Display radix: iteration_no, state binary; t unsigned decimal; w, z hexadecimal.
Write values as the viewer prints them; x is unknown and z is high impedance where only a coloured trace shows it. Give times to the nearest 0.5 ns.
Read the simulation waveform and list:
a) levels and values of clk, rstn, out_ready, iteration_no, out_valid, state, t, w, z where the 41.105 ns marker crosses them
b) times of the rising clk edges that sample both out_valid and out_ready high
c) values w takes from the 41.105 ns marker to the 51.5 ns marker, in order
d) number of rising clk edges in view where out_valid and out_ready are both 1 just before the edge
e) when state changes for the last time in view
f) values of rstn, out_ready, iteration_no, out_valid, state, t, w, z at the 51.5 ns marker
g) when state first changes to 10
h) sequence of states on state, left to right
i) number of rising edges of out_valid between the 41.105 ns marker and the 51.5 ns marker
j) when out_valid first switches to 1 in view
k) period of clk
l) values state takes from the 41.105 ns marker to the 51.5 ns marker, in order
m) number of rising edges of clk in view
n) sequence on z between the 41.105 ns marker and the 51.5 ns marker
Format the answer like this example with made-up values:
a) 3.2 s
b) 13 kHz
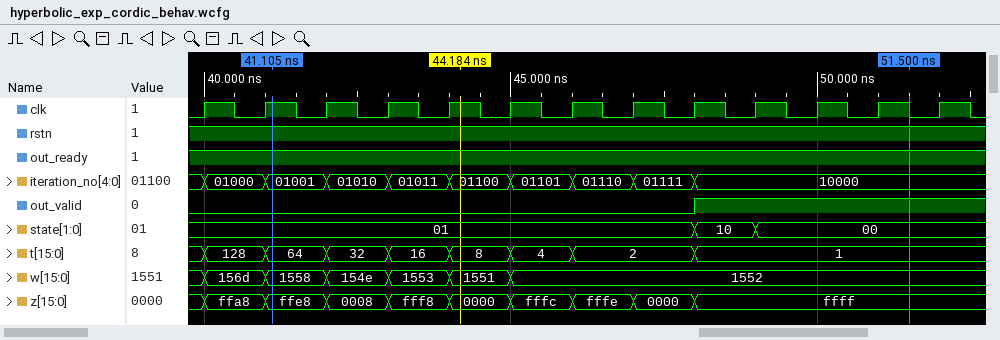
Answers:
a) clk=1, rstn=1, out_ready=1, iteration_no=01001, out_valid=0, state=01, t=64, w=1558, z=ffe8
b) 49 ns, 50 ns, 51 ns, 52 ns
c) 1558, 154e, 1553, 1551, 1552
d) 4
e) 49 ns
f) rstn=1, out_ready=1, iteration_no=10000, out_valid=1, state=00, t=1, w=1552, z=ffff
g) 48 ns
h) 01, 10, 00
i) 1
j) 48 ns
k) 1 ns
l) 01, 10, 00
m) 13
n) ffe8, 0008, fff8, 0000, fffc, fffe, 0000, ffff
